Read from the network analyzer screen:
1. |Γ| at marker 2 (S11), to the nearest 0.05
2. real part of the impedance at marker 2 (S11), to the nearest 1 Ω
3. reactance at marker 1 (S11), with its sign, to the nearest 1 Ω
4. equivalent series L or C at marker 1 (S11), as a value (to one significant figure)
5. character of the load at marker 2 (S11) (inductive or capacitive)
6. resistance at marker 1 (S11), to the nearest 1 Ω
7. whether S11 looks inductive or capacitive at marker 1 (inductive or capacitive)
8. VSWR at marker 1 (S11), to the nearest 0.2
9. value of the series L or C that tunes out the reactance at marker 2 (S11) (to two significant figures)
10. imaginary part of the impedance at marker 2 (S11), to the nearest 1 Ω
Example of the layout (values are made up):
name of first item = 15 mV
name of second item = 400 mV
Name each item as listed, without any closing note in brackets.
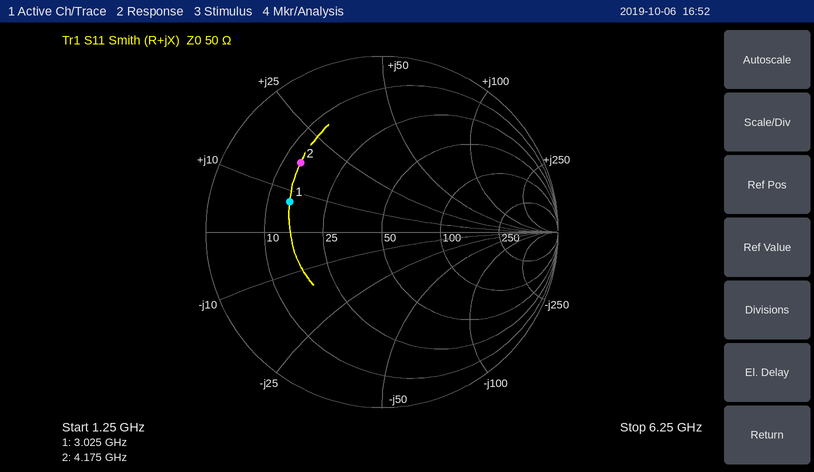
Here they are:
|Γ| at marker 2 (S11), to the nearest 0.05 = 0.60
real part of the impedance at marker 2 (S11), to the nearest 1 Ω = 14 Ω
reactance at marker 1 (S11), with its sign, to the nearest 1 Ω = +7 Ω
equivalent series L or C at marker 1 (S11), as a value = 400 pH
character of the load at marker 2 (S11) = inductive
resistance at marker 1 (S11), to the nearest 1 Ω = 15 Ω
whether S11 looks inductive or capacitive at marker 1 = inductive
VSWR at marker 1 (S11), to the nearest 0.2 = 3.4
value of the series L or C that tunes out the reactance at marker 2 (S11) = 2.2 pF
imaginary part of the impedance at marker 2 (S11), to the nearest 1 Ω = +17 Ω
